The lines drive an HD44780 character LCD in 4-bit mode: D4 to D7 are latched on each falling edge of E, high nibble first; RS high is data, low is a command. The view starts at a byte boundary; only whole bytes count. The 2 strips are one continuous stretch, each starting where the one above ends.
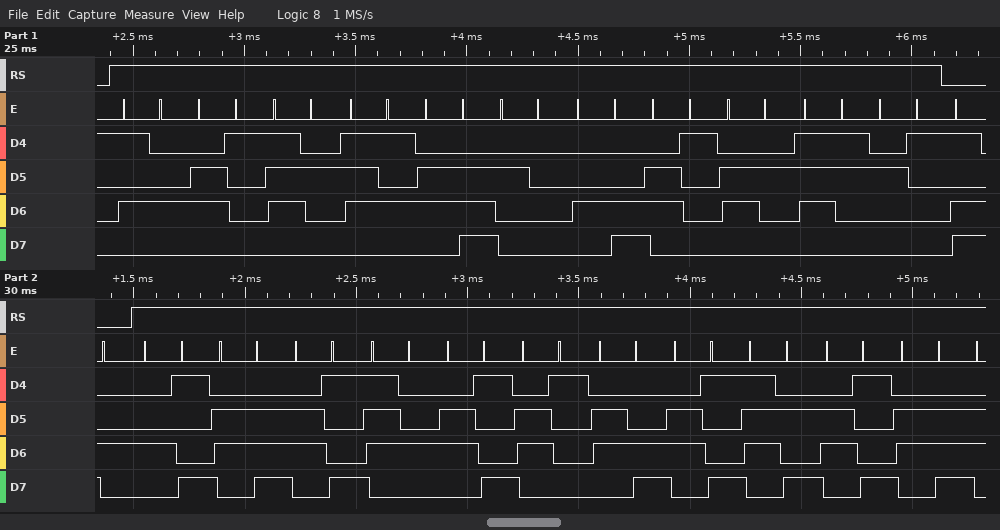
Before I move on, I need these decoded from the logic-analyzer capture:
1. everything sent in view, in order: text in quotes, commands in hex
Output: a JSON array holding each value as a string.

["\"Tarun Labs!\" 0xD4 \"Initializin\""]
